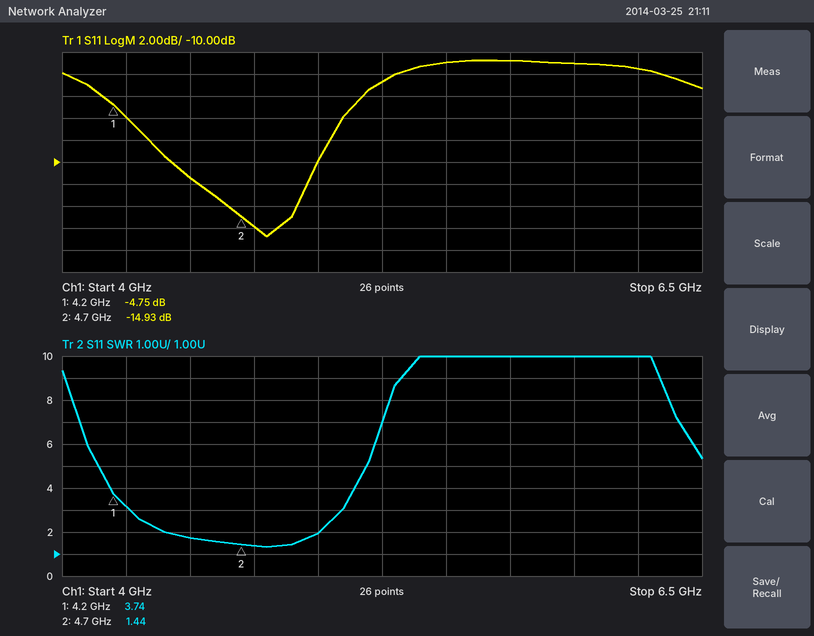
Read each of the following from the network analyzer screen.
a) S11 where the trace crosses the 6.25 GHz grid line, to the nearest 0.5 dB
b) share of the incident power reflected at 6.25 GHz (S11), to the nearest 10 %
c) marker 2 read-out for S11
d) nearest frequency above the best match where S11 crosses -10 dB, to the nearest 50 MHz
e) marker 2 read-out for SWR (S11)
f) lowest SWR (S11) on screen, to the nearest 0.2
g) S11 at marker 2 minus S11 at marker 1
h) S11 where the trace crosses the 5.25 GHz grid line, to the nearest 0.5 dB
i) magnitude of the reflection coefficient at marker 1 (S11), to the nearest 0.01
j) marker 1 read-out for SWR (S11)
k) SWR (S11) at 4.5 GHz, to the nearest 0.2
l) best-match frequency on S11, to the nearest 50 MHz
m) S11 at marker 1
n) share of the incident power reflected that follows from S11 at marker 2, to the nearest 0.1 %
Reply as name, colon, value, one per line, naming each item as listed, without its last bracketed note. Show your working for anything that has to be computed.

S11 where the trace crosses the 6.25 GHz grid line, to the nearest 0.5 dB: -1.5 dB
share of the incident power reflected at 6.25 GHz (S11), to the nearest 10 %: 10^(-1.5/10) ≈ 70.8 %, so 70 % to the nearest 10 %
marker 2 read-out for S11: -14.93 dB
nearest frequency above the best match where S11 crosses -10 dB, to the nearest 50 MHz: 5.00 GHz
marker 2 read-out for SWR: 1.44
lowest SWR (S11) on screen, to the nearest 0.2: 1.4
S11 at marker 2 minus S11 at marker 1: -14.93 − (-4.75) = -10.18 dB
S11 where the trace crosses the 5.25 GHz grid line, to the nearest 0.5 dB: -2.5 dB
magnitude of the reflection coefficient at marker 1 (S11), to the nearest 0.01: 10^(-4.75/20) ≈ 0.58
marker 1 read-out for SWR: 3.74
SWR (S11) at 4.5 GHz, to the nearest 0.2: 1.8
best-match frequency on S11, to the nearest 50 MHz: 4.80 GHz
S11 at marker 1: -4.75 dB
share of the incident power reflected that follows from S11 at marker 2, to the nearest 0.1 %: 10^(-14.93/10) ≈ 3.2 %
